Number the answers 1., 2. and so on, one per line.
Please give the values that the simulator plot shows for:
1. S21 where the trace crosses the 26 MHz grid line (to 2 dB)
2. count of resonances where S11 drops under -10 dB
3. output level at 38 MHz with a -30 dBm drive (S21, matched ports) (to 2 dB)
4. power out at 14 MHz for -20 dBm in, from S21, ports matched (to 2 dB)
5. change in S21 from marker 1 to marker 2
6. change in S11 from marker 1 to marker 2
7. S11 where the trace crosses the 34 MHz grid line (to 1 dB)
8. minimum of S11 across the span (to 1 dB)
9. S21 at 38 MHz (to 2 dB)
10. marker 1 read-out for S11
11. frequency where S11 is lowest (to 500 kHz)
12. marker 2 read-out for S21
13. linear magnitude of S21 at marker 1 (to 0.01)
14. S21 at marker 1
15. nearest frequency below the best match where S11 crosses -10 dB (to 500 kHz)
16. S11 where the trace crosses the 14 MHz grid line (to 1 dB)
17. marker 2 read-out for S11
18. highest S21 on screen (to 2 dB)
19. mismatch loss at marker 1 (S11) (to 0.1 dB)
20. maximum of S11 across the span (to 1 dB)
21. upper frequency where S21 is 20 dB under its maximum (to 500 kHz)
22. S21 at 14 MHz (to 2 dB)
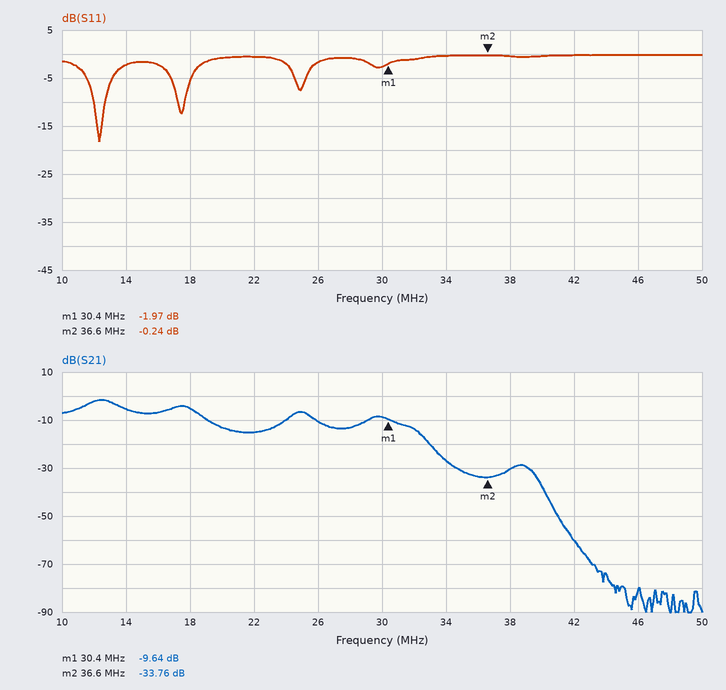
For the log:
1. -10 dB
2. 2
3. -60 dBm
4. -26 dBm
5. -24.12 dB
6. 1.73 dB
7. 0 dB
8. -18 dB
9. -30 dB
10. -1.97 dB
11. 12.5 MHz
12. -33.76 dB
13. 0.33
14. -9.64 dB
15. 12.0 MHz
16. -2 dB
17. -0.24 dB
18. -2 dB
19. 4.4 dB
20. 0 dB
21. 33.0 MHz
22. -6 dB
